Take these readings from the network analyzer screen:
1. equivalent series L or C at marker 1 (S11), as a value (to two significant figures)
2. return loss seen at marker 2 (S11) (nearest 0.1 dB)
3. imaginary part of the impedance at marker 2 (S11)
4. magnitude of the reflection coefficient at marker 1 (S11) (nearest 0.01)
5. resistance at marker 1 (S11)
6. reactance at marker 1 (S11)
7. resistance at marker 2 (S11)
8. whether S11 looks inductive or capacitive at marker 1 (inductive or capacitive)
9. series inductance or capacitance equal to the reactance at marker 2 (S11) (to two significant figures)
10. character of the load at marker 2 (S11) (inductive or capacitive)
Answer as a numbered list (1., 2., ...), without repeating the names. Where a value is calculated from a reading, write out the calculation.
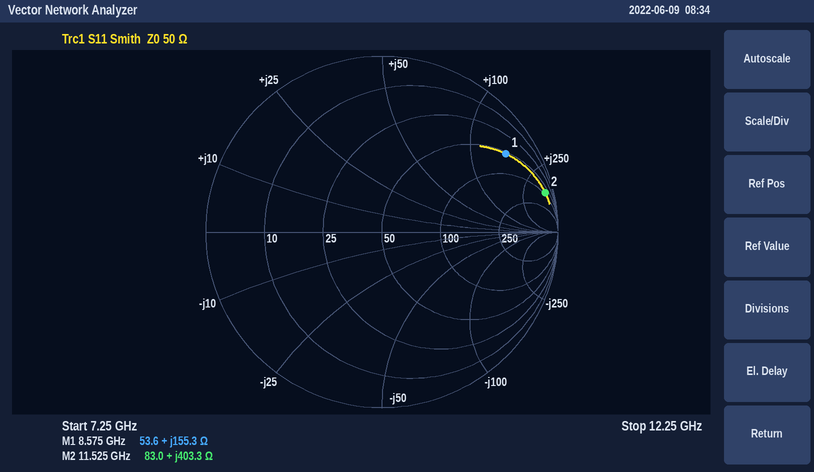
1. L = 155.3 Ω/(2π × 8.575 GHz) ≈ 2.9 nH
2. 0.4 dB
3. +403.3 Ω
4. 0.83
5. 53.6 Ω
6. +155.3 Ω
7. 83.0 Ω
8. inductive
9. L = 403.3 Ω/(2π × 11.525 GHz) ≈ 5.6 nH
10. inductive
